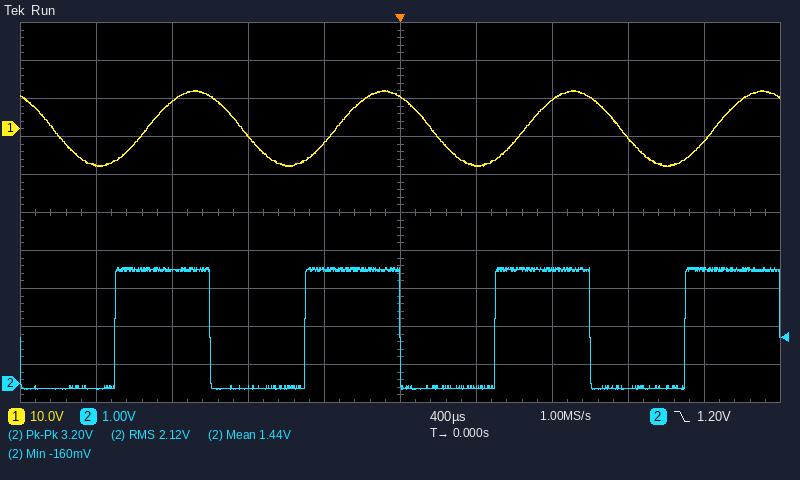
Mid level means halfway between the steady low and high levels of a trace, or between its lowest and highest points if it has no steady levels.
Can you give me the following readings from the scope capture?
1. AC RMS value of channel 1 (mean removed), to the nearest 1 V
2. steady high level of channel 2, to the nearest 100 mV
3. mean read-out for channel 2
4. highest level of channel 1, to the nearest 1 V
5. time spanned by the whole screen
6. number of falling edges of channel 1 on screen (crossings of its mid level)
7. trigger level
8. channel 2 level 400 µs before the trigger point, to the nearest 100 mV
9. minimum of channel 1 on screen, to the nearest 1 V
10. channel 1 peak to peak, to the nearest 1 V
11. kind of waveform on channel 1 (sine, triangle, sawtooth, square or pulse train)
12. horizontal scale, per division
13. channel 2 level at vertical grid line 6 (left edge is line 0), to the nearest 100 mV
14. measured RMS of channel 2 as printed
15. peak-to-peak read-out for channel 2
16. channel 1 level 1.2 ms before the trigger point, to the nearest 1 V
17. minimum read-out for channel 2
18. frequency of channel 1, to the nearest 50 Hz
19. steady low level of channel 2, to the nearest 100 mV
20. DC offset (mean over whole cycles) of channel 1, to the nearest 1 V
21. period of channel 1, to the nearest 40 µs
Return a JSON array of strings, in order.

["7 V", "3.0 V", "1.44 V", "10 V", "4 ms", "4", "1.20 V", "3.0 V", "-10 V", "20 V", "sine", "400 µs", "-100 mV", "2.12 V", "3.20 V", "7 V", "-160 mV", "1.00 kHz", "-100 mV", "0 V", "1.00 ms"]
